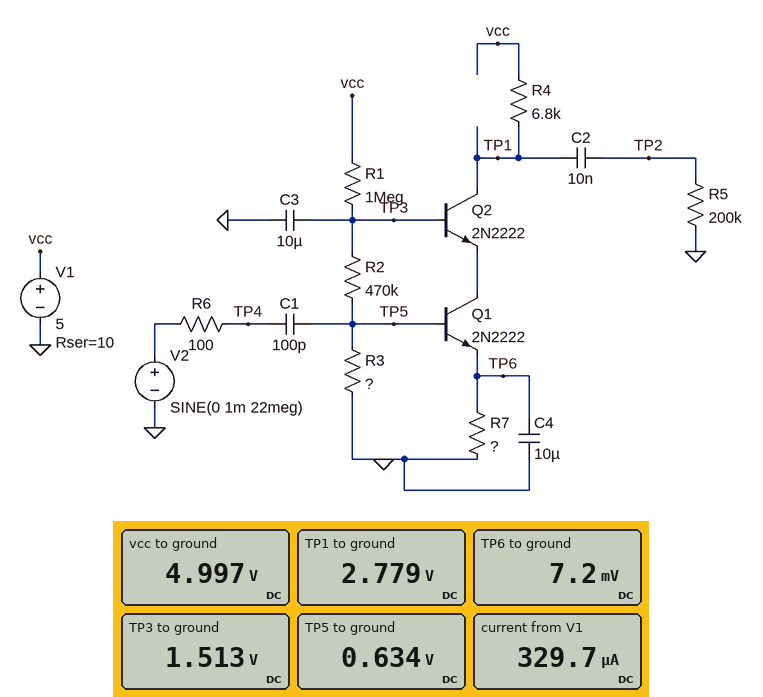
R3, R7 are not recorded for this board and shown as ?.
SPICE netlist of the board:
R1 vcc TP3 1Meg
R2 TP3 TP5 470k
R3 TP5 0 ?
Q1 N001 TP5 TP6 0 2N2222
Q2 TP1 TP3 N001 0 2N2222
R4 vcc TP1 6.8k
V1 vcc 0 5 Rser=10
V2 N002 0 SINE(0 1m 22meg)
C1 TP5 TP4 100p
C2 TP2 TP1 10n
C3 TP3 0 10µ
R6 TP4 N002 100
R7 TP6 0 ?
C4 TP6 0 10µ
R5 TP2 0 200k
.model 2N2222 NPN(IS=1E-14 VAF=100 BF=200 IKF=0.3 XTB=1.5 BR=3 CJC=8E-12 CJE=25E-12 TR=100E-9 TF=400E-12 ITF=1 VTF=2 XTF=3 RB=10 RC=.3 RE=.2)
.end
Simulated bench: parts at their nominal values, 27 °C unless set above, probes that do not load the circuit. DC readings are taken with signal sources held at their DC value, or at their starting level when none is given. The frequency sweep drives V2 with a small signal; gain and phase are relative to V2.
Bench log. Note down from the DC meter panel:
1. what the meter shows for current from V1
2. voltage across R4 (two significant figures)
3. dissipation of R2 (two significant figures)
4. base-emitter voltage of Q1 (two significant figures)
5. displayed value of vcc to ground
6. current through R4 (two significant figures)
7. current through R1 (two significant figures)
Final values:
329.7 µA
2.2 V
1.6 µW
630 mV
4.997 V
330 µA
3.5 µA
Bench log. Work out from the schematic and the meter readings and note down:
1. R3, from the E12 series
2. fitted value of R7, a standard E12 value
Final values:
2.7 MΩ
22 Ω
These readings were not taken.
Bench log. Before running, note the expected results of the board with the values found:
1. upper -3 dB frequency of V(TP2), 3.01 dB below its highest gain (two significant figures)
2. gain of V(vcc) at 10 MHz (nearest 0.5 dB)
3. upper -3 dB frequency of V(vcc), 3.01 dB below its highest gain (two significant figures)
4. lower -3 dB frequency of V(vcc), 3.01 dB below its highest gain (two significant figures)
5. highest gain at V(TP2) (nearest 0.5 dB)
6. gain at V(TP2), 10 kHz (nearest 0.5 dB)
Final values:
4.2 MHz
-31.0 dB
4.2 MHz
64 kHz
34.0 dB
18.0 dB
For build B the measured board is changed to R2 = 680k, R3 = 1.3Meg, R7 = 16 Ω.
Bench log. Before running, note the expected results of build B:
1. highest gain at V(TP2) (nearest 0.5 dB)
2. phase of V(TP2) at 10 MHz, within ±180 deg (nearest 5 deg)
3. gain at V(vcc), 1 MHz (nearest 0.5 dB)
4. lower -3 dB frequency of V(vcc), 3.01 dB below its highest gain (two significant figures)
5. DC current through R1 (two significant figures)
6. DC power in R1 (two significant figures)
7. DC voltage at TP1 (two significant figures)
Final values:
32.5 dB
80 deg
-24.0 dB
54 kHz
3.1 µA
9.8 µW
3.2 V
